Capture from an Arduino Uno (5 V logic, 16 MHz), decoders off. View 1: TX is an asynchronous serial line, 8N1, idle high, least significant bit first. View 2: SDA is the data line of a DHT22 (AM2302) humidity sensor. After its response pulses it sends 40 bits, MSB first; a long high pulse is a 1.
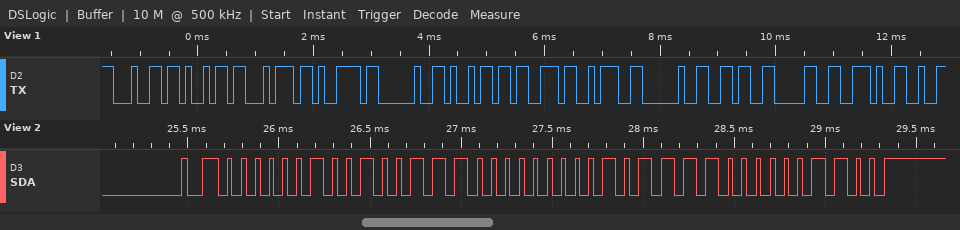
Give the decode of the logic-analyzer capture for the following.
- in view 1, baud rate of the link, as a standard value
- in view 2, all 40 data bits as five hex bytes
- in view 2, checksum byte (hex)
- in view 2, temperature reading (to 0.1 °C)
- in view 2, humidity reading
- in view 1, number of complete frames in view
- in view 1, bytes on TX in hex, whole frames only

9600 baud
02 4E 00 BC 0C
0x0C
18.8 °C
59.0 %
12
64 69 74 79 20 69 73 3A 20 36 30 2E
